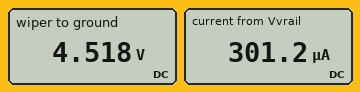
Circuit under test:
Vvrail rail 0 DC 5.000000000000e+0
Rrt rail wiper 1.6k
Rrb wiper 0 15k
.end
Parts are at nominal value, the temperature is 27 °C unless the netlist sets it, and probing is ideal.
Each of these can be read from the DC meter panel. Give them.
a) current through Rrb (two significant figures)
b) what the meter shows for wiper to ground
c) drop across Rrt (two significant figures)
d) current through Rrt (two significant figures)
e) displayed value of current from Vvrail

300 µA
4.518 V
480 mV
300 µA
301.2 µA
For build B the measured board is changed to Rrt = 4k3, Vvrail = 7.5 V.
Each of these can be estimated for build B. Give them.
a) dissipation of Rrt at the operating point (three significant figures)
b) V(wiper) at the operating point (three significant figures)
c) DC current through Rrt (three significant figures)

649 µW
5.83 V
389 µA
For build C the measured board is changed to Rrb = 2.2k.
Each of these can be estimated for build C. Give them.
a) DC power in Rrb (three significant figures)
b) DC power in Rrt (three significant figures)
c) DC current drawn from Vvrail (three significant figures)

3.81 mW
2.77 mW
1.32 mA
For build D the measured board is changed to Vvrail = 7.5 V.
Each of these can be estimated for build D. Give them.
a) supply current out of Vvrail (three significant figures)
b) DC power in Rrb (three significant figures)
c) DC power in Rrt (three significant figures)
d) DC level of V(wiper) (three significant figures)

452 µA
3.06 mW
327 µW
6.78 V
